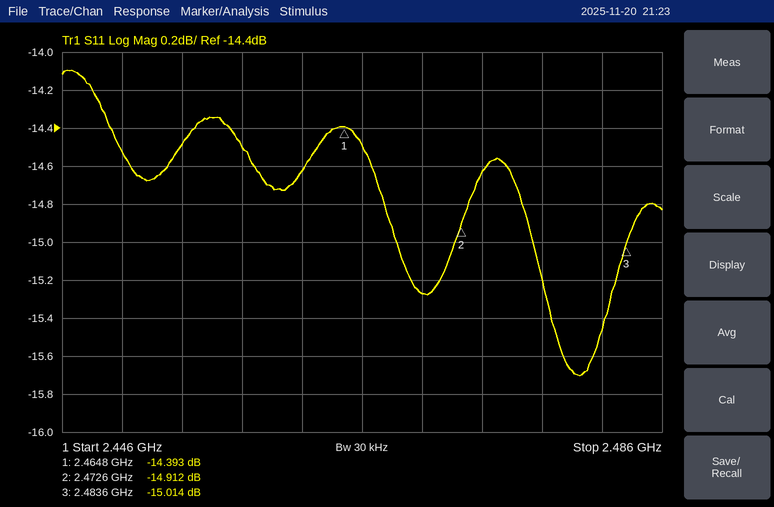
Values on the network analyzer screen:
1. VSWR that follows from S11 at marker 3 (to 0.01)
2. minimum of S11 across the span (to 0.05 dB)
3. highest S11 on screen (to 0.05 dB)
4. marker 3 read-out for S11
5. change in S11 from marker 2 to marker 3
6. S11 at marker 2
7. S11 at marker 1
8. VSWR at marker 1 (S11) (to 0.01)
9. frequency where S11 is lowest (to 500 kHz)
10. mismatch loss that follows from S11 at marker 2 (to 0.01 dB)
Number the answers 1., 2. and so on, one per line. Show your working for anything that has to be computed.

1. (1 + 0.1775)/(1 − 0.1775) ≈ 1.43
2. -15.70 dB
3. -14.10 dB
4. -15.014 dB
5. -15.014 − (-14.912) = -0.102 dB
6. -14.912 dB
7. -14.393 dB
8. (1 + 0.1907)/(1 − 0.1907) ≈ 1.47
9. 2.4805 GHz
10. −10 log10(1 − 10^(-14.912/10)) ≈ 0.14 dB
